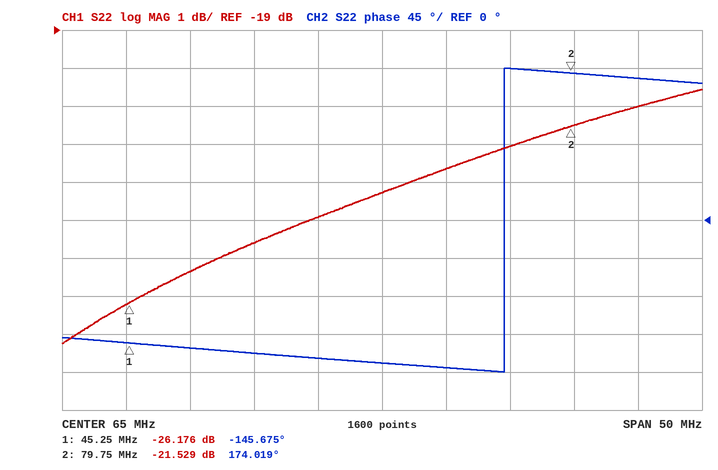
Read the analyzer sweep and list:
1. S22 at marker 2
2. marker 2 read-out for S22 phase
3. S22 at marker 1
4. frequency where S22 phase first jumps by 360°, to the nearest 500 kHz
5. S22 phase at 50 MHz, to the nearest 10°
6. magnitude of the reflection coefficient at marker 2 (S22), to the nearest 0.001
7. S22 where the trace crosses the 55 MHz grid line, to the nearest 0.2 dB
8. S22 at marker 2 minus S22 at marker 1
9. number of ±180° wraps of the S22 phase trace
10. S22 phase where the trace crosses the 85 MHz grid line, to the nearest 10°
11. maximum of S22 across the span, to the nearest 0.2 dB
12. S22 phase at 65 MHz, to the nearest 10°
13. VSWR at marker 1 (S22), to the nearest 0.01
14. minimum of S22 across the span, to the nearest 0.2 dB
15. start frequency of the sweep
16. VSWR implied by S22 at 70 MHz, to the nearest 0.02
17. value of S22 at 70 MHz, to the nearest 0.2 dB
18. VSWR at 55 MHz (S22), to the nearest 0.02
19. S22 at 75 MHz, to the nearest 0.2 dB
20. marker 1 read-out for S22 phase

-21.529 dB
174.019°
-26.176 dB
74.5 MHz
-150°
0.084
-24.6 dB
4.647 dB
1
170°
-20.6 dB
-170°
1.10
-27.2 dB
40 MHz
1.16
-22.6 dB
1.12
-22.0 dB
-145.675°
